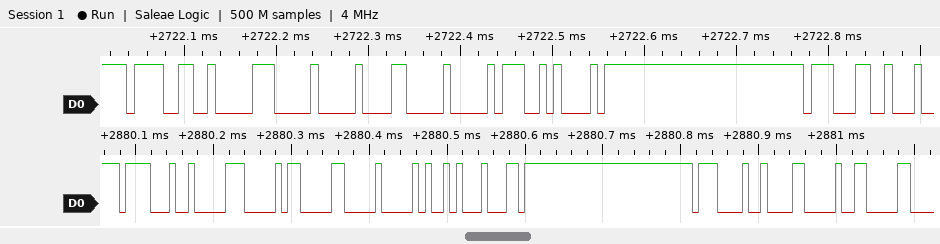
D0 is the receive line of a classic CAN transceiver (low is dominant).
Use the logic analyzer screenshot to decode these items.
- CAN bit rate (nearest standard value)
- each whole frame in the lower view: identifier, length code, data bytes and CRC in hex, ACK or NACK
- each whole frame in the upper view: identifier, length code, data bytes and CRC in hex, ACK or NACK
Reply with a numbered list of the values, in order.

1. 125 kbit/s
2. ID 789, DLC 3, data 03 04 00, CRC 2511, ACK
3. ID 799, DLC 3, data 00 03 00, CRC 0E50, ACK
